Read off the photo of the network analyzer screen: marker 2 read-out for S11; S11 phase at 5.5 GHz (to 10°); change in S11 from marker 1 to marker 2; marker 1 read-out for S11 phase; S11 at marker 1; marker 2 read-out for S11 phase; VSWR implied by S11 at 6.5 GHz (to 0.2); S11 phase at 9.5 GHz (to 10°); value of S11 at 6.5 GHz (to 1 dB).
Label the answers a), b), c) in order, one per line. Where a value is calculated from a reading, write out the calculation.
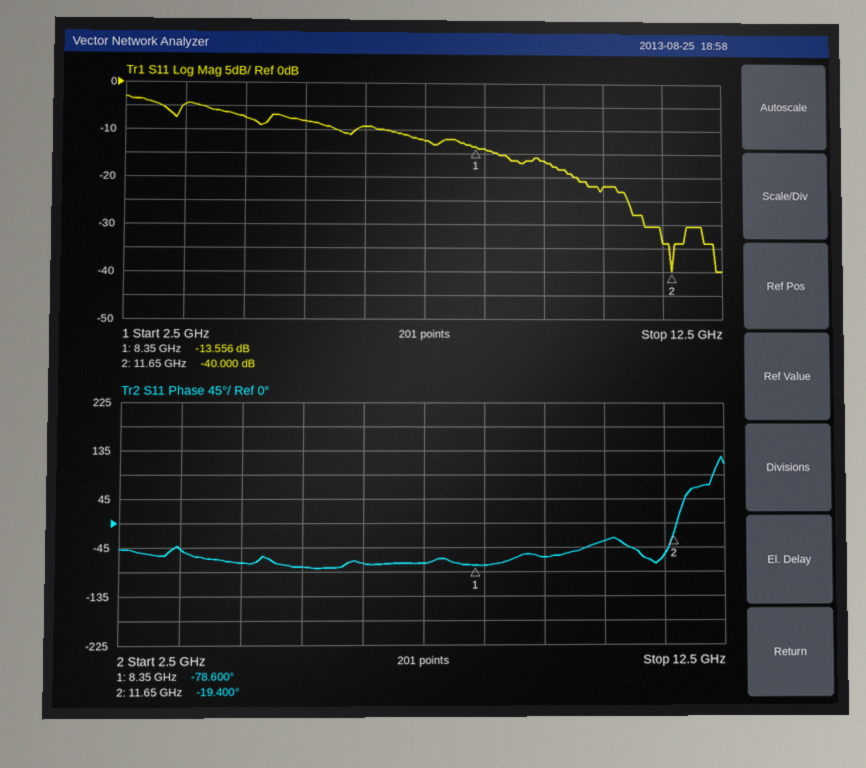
a) -40.000 dB
b) -80°
c) -40 − (-13.556) = -26.444 dB
d) -78.600°
e) -13.556 dB
f) -19.400°
g) |Γ| = 10^(-9/20) = 0.3548; VSWR = (1 + 0.3548)/(1 − 0.3548) ≈ 2.10, so 2.0 to the nearest 0.2
h) -60°
i) -9 dB
